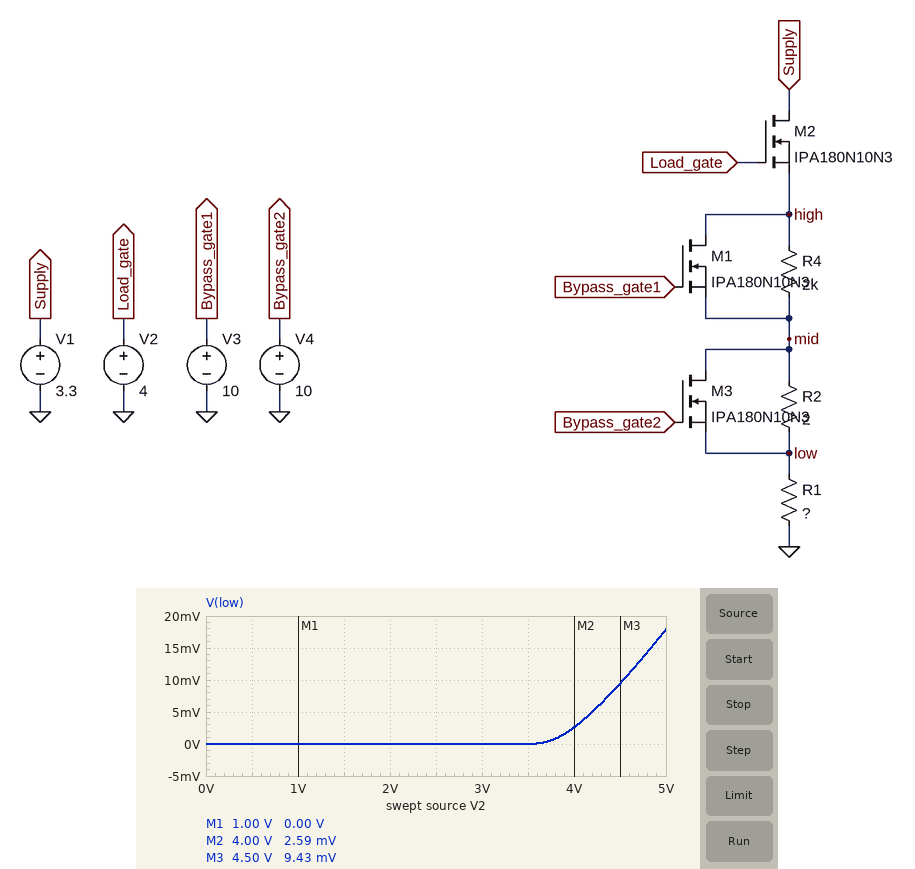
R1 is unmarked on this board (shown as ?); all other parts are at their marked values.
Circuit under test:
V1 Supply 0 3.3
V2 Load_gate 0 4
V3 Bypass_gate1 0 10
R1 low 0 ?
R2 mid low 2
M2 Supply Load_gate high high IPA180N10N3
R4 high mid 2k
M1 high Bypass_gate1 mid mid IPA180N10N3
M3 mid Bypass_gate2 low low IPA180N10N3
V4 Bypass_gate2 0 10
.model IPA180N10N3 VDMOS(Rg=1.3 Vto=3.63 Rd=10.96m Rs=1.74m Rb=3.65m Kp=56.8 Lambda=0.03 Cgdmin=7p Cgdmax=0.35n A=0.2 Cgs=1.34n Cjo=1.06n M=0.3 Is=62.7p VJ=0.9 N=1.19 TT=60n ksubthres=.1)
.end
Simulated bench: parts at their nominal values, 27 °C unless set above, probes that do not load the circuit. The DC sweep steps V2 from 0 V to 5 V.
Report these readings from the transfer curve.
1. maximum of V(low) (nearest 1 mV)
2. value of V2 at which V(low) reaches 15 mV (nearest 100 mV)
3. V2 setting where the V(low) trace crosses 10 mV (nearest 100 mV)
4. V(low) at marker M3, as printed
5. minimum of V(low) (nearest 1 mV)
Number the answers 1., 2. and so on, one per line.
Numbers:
1. 18 mV
2. 4.8 V
3. 4.5 V
4. 9.43 mV
5. 0 V
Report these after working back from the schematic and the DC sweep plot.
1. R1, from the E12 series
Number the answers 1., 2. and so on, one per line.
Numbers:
1. 1 mΩ
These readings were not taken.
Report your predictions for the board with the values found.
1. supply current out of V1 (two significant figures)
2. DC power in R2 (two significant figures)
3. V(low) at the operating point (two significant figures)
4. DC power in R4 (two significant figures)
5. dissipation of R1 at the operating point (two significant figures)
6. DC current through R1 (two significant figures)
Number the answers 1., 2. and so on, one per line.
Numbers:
1. 2.6 A
2. 790 µW
3. 2.6 mV
4. 810 nW
5. 6.7 mW
6. 2.6 A
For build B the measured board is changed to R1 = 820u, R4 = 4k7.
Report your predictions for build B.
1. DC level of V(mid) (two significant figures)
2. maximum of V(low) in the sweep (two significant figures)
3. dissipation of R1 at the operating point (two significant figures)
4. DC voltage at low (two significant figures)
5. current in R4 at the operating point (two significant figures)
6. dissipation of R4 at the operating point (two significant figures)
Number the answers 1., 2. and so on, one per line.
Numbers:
1. 42 mV
2. 15 mV
3. 5.5 mW
4. 2.1 mV
5. 8.6 µA
6. 340 nW
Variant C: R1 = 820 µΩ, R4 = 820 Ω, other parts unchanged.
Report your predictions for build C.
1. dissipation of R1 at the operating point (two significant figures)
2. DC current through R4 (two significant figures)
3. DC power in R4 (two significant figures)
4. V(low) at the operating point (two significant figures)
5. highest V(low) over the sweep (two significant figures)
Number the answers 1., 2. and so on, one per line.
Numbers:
1. 5.5 mW
2. 49 µA
3. 2.0 µW
4. 2.1 mV
5. 15 mV
